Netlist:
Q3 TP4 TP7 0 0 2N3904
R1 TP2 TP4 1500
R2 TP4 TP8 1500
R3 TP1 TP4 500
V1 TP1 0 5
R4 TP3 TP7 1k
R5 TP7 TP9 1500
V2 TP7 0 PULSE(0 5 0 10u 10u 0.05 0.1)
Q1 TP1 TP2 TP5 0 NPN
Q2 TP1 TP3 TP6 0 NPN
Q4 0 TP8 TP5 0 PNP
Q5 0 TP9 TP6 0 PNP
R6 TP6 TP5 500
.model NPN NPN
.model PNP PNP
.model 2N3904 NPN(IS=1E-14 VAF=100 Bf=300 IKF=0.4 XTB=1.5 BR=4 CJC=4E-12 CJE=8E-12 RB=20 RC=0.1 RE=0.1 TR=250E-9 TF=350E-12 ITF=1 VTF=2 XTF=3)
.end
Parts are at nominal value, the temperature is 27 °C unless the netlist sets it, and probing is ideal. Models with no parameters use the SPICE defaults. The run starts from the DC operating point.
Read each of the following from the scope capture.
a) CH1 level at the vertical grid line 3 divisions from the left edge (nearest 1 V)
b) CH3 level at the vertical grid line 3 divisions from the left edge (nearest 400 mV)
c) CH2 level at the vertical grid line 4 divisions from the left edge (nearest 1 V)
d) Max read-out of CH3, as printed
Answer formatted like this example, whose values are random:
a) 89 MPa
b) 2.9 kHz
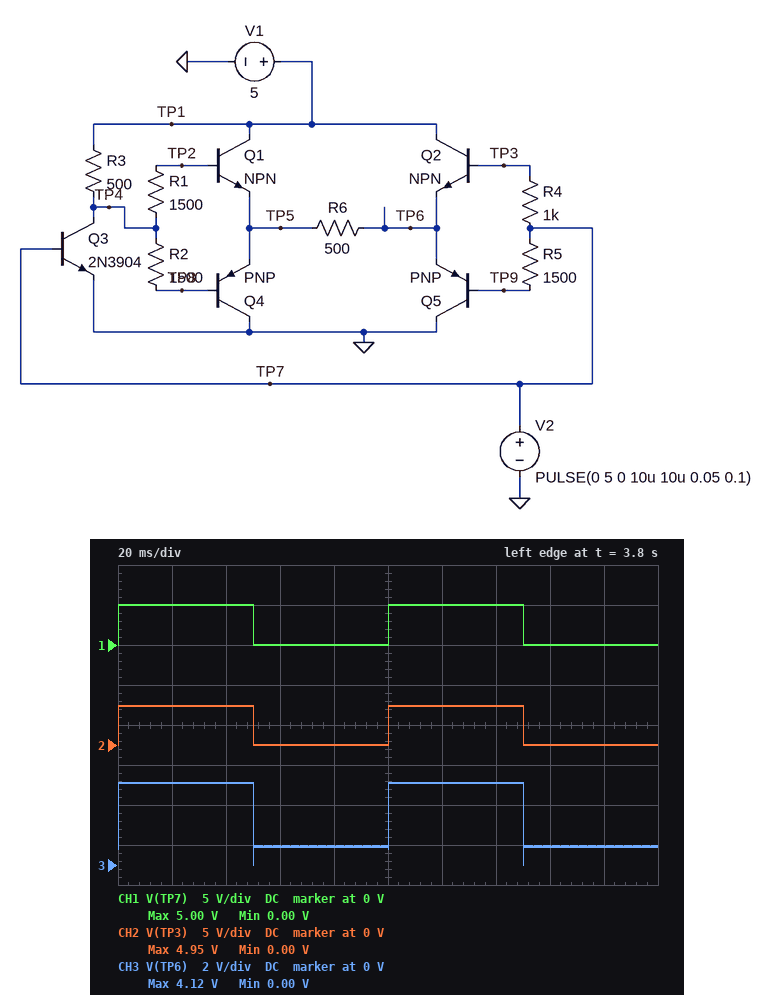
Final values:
a) 0 V
b) 800 mV
c) 0 V
d) 4.12 V
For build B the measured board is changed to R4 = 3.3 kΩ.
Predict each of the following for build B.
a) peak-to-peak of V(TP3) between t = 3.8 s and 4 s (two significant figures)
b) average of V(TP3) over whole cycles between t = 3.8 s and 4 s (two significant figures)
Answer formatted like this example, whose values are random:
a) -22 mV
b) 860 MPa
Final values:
a) 4.8 V
b) 2.4 V
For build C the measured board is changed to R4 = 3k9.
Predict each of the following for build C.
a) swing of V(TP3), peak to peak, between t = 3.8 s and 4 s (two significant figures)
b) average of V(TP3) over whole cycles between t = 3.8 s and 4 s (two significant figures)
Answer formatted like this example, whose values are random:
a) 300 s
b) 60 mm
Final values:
a) 4.8 V
b) 2.4 V
